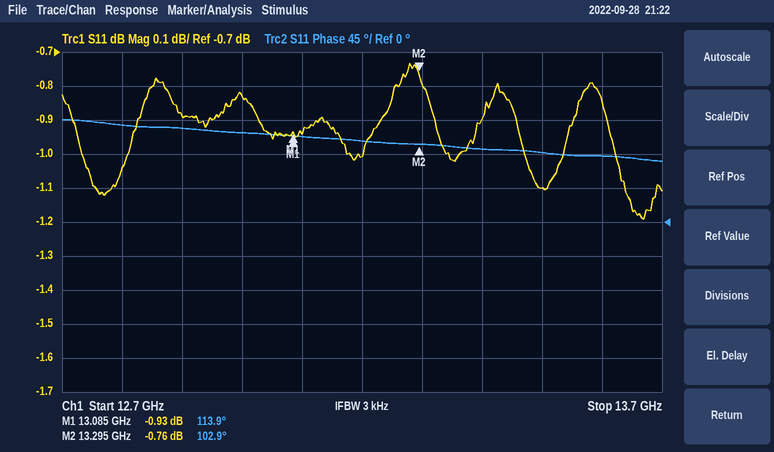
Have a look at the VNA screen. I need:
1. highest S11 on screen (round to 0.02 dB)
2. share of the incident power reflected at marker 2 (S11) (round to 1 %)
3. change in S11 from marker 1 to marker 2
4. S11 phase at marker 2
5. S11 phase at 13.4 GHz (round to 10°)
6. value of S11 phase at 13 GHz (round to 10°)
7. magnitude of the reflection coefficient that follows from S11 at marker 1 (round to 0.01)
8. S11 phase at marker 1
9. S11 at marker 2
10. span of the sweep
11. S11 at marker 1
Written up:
-0.74 dB
84 %
0.17 dB
102.9°
100°
120°
0.90
113.9°
-0.76 dB
1 GHz
-0.93 dB
